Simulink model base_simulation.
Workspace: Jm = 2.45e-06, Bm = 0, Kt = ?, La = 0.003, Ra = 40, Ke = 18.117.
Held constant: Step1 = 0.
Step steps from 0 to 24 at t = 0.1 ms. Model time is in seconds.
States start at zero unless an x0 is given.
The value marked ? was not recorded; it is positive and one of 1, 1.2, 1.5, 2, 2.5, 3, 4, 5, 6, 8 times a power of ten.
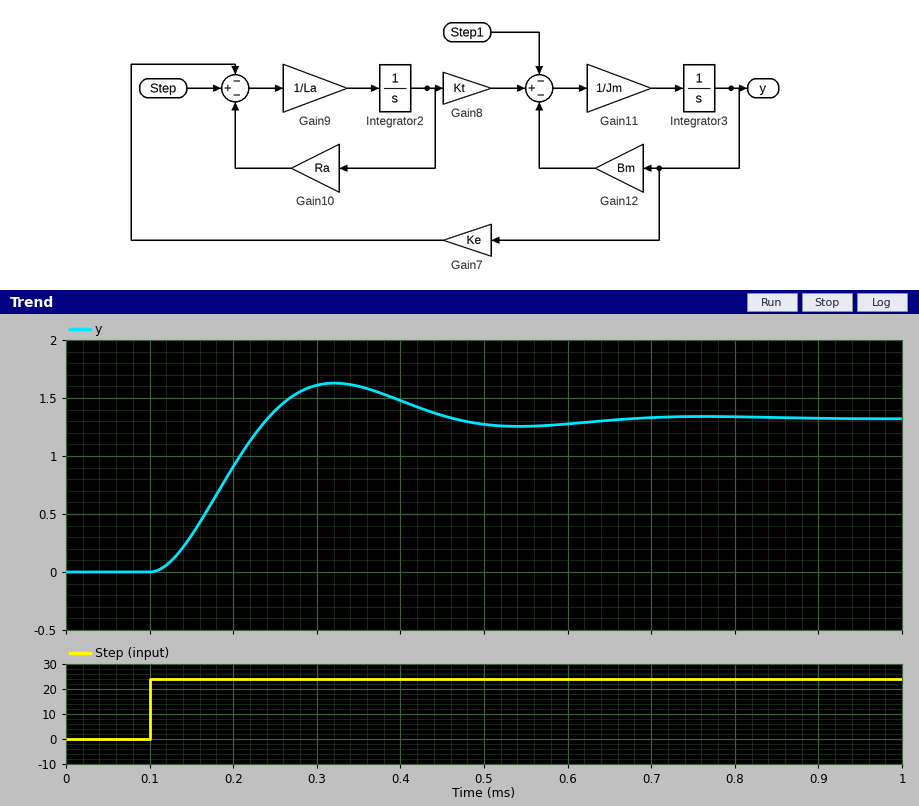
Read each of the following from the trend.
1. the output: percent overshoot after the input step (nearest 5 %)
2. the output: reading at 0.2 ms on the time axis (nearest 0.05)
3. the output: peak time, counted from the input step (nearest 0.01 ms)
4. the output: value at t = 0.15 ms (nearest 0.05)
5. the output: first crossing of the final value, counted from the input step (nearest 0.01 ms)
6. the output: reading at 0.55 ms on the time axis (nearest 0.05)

25 %
0.90
0.22 ms
0.30
0.14 ms
1.25
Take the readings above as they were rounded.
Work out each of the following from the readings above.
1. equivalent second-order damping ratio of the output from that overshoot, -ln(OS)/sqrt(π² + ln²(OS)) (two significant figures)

0.40
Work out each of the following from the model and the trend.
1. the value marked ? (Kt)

0.1
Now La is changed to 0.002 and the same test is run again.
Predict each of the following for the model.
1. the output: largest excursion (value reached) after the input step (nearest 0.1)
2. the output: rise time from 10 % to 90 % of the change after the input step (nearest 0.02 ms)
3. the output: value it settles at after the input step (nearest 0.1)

1.5
0.08 ms
1.3
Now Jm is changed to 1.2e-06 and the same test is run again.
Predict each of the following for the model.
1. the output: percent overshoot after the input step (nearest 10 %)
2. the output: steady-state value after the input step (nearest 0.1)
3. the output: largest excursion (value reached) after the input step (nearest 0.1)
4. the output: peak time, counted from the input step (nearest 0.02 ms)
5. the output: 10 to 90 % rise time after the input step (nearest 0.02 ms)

40 %
1.3
1.8
0.14 ms
0.06 ms
